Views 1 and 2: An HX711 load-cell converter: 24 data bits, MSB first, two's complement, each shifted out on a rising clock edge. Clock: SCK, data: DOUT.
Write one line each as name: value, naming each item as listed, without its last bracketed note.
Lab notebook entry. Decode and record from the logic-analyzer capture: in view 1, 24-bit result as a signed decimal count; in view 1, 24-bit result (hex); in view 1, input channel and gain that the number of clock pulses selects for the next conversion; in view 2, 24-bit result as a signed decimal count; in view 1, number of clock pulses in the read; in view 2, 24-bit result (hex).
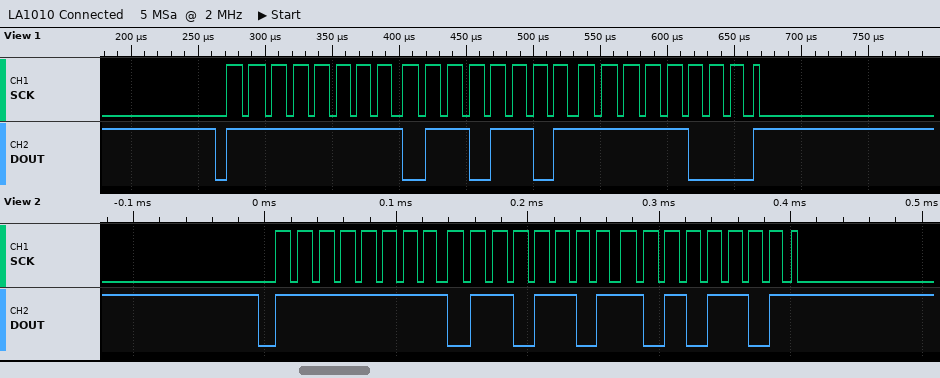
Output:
in view 1, 24-bit result as a signed decimal count: -37384
in view 1, 24-bit result: 0xFF6DF8
in view 1, input channel and gain that the number of clock pulses selects for the next conversion: channel A, gain 128
in view 2, 24-bit result as a signed decimal count: -37459
in view 1, number of clock pulses in the read: 25
in view 2, 24-bit result: 0xFF6DAD
